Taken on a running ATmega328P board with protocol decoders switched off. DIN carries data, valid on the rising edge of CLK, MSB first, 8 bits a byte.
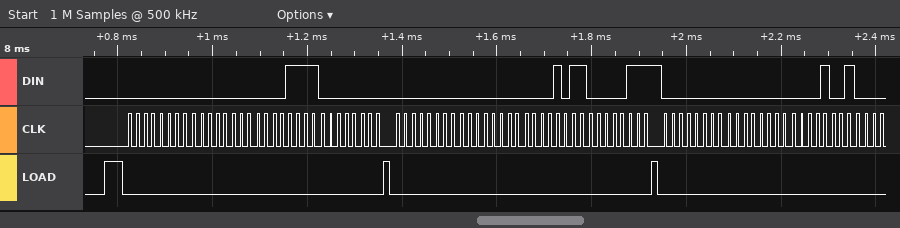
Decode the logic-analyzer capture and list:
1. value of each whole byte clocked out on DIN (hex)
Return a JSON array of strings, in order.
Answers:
["00 00 0F 00 00 00 0B 07 00 00 09"]
